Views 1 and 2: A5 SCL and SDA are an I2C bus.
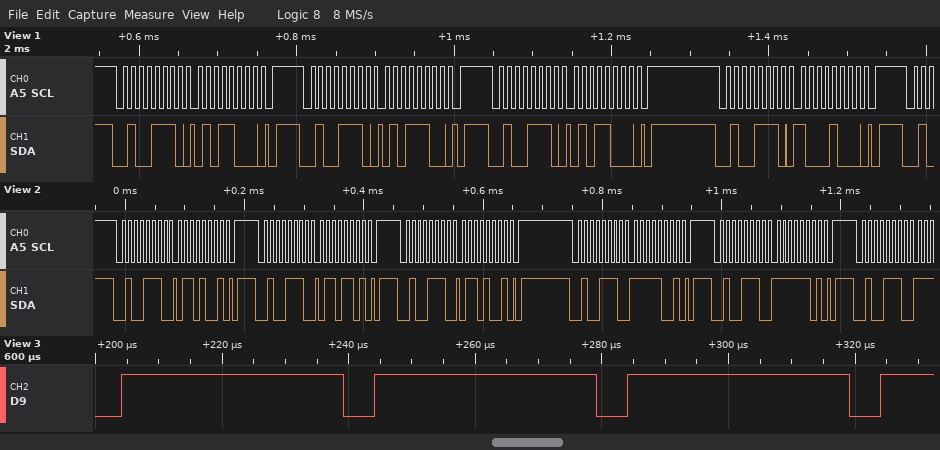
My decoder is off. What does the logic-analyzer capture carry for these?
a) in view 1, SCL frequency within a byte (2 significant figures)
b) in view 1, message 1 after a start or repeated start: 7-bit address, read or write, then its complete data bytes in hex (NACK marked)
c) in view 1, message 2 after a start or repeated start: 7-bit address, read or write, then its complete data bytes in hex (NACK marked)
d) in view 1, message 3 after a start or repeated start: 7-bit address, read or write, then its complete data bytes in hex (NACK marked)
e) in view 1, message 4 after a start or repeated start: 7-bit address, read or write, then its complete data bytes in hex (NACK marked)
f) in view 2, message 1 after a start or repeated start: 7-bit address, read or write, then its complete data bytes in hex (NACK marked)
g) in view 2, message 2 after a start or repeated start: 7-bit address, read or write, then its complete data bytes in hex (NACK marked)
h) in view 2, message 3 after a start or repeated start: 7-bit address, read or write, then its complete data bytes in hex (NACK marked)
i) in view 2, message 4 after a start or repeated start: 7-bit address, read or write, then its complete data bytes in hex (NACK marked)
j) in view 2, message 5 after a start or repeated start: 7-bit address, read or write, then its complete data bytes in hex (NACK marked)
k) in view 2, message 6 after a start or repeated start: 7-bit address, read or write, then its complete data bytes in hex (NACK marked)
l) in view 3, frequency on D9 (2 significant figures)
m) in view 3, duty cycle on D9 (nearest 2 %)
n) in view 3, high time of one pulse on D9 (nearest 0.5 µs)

100 kHz
0x27 write: 58
0x27 write: 5C
0x27 write: 58
0x27 write: 88
0x27 write: 69
0x27 write: 6D
0x27 write: 69
0x27 write: F9
0x27 write: FD
0x27 write
25 kHz
88 %
35.0 µs
